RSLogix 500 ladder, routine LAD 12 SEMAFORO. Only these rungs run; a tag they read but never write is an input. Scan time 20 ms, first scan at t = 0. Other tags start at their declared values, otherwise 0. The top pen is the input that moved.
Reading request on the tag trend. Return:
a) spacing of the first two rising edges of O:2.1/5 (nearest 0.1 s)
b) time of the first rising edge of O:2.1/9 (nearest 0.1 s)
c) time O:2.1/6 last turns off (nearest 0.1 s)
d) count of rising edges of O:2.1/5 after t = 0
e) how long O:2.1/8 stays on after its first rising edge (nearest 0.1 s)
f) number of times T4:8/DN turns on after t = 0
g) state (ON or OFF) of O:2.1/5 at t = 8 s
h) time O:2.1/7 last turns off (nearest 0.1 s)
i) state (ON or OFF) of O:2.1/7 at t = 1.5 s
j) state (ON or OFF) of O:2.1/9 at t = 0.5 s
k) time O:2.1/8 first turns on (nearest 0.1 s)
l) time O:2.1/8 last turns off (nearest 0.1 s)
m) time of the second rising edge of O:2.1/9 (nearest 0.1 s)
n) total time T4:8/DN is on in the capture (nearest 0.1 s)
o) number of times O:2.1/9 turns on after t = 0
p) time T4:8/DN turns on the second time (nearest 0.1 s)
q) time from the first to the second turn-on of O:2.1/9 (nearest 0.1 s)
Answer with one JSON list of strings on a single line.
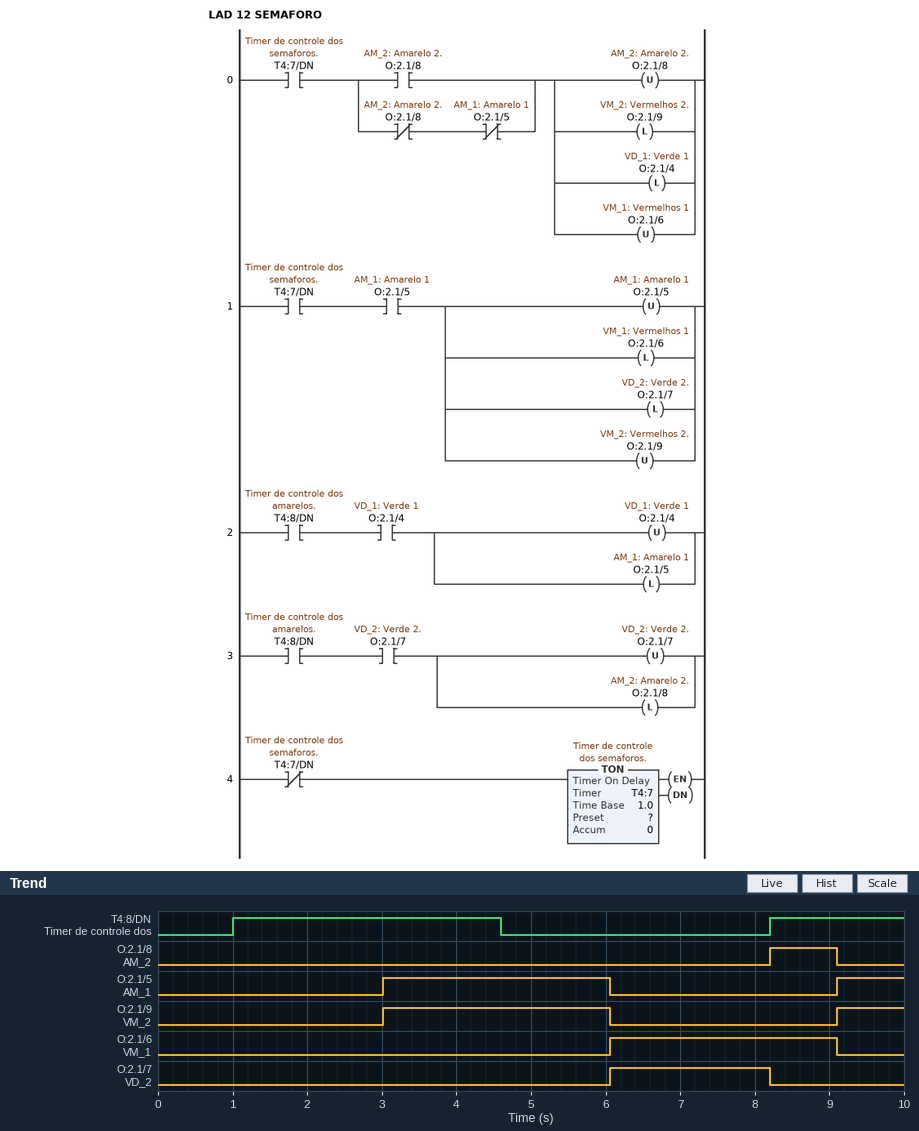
["6.1 s", "3.0 s", "9.1 s", "2", "0.9 s", "2", "OFF", "8.2 s", "OFF", "OFF", "8.2 s", "9.1 s", "9.1 s", "5.4 s", "2", "8.2 s", "6.1 s"]
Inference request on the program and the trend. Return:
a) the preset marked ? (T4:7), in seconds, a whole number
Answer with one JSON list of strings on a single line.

["3 s"]
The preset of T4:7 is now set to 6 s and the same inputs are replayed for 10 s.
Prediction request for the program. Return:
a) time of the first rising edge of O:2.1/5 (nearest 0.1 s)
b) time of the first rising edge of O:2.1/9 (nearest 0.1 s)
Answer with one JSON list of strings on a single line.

["8.2 s", "6.0 s"]
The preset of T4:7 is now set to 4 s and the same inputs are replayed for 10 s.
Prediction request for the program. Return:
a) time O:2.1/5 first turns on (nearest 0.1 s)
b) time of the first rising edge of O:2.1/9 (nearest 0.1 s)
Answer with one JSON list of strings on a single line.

["4.0 s", "4.0 s"]
